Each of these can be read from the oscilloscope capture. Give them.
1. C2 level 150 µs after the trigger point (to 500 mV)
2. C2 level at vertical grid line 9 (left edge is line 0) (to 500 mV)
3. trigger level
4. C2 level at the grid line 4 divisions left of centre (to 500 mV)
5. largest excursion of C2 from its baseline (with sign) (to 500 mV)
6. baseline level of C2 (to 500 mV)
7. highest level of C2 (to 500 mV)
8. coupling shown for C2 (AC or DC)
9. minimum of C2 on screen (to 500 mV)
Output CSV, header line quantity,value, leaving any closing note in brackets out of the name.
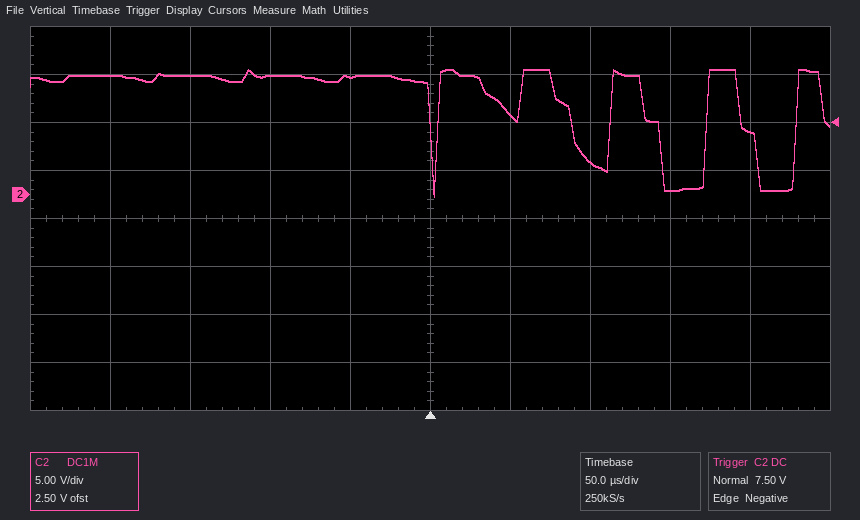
quantity,value
C2 level 150 µs after the trigger point,500 mV
C2 level at vertical grid line 9 (left edge is line 0),6.5 V
trigger level,7.50 V
C2 level at the grid line 4 divisions left of centre,12.5 V
largest excursion of C2 from its baseline (with sign),-12.5 V
baseline level of C2,12.5 V
highest level of C2,13.0 V
coupling shown for C2,DC
minimum of C2 on screen,0.0 V
